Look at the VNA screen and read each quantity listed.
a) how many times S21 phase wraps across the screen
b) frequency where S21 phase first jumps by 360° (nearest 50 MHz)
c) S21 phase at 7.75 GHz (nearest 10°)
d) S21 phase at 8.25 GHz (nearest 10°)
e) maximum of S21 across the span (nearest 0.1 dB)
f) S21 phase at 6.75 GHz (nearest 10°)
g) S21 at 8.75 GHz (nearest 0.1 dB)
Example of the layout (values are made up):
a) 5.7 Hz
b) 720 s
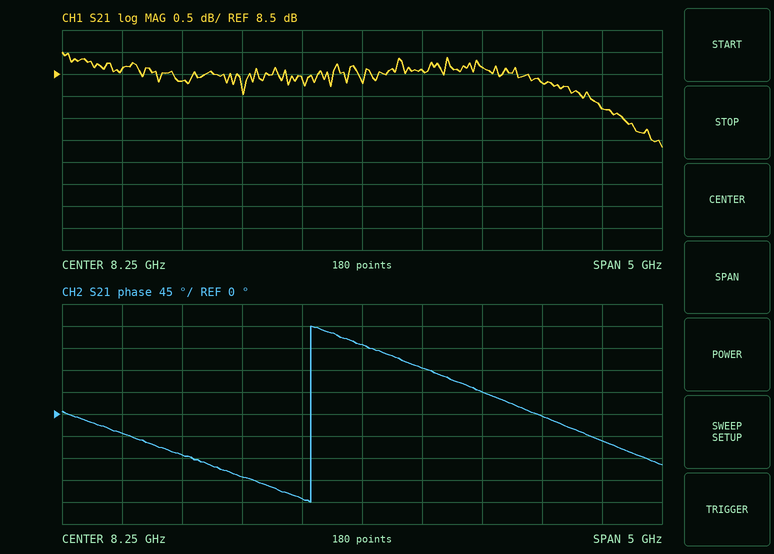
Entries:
a) 1
b) 7.80 GHz
c) -170°
d) 140°
e) 9.0 dB
f) -80°
g) 8.6 dB
